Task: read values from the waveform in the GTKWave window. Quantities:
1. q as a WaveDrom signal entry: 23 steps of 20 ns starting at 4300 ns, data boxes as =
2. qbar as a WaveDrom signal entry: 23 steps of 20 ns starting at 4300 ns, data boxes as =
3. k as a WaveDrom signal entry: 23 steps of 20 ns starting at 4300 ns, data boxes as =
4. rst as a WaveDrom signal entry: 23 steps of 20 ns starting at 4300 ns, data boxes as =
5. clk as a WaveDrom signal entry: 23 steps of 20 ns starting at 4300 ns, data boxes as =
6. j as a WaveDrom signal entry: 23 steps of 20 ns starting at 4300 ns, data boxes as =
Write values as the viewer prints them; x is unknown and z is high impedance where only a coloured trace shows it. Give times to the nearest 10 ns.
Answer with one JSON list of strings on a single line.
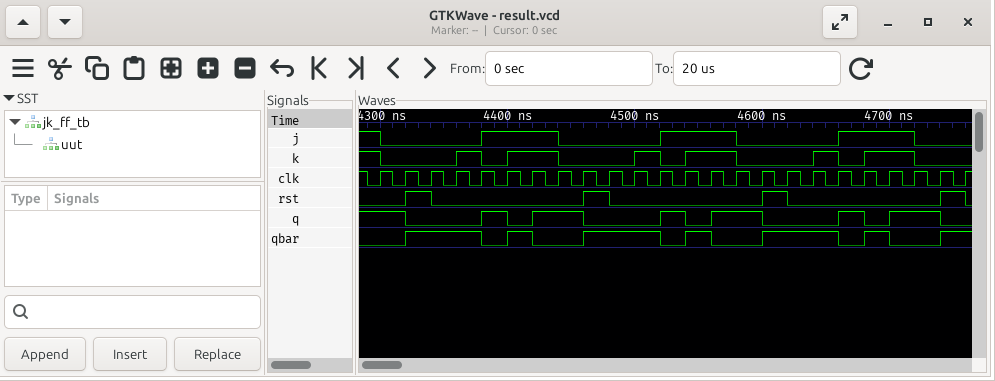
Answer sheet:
["{name: 'q', wave: '10..101.0..101.0..101.0'}", "{name: 'qbar', wave: '01..010.1..010.1..010.1'}", "{name: 'k', wave: '0..101.0..101.0..101.0.'}", "{name: 'rst', wave: '010.....10.....10.....1'}", "{name: 'clk', wave: 'p......................'}", "{name: 'j', wave: '0...1..0...1..0...1..0.'}"]
